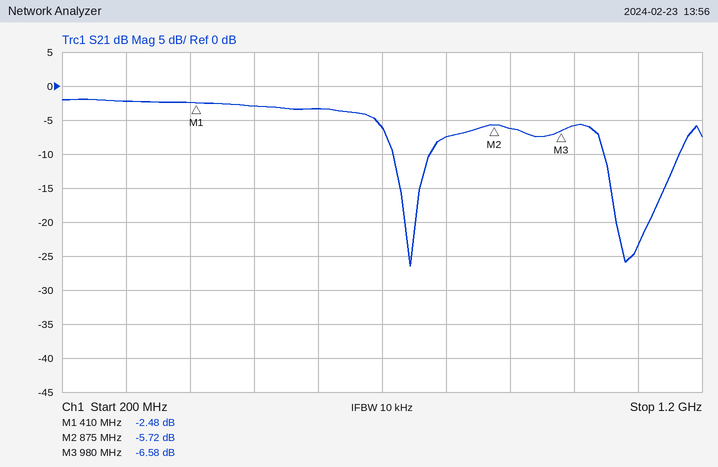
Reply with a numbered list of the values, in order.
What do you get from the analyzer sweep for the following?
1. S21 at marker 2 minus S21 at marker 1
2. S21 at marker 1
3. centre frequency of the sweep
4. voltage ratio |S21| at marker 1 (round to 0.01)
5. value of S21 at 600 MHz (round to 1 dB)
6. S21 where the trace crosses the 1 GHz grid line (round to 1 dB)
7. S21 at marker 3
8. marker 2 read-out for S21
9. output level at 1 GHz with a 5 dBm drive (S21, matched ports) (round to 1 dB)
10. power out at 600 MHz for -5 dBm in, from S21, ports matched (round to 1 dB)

1. -3.24 dB
2. -2.48 dB
3. 700 MHz
4. 0.75
5. -3 dB
6. -6 dB
7. -6.58 dB
8. -5.72 dB
9. -1 dBm
10. -8 dBm
